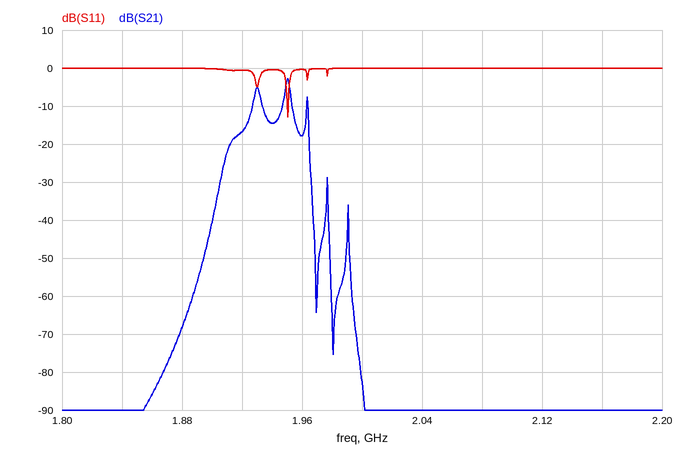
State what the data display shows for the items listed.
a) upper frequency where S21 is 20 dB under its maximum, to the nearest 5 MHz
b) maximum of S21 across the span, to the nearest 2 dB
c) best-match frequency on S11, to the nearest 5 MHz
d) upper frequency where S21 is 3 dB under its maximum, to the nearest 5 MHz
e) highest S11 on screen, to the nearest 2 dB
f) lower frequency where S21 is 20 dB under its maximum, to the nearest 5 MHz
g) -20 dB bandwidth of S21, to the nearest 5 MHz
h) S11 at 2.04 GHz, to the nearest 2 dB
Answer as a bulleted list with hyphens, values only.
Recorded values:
- 1.965 GHz
- -2 dB
- 1.950 GHz
- 1.950 GHz
- 0 dB
- 1.910 GHz
- 55 MHz
- 0 dB
